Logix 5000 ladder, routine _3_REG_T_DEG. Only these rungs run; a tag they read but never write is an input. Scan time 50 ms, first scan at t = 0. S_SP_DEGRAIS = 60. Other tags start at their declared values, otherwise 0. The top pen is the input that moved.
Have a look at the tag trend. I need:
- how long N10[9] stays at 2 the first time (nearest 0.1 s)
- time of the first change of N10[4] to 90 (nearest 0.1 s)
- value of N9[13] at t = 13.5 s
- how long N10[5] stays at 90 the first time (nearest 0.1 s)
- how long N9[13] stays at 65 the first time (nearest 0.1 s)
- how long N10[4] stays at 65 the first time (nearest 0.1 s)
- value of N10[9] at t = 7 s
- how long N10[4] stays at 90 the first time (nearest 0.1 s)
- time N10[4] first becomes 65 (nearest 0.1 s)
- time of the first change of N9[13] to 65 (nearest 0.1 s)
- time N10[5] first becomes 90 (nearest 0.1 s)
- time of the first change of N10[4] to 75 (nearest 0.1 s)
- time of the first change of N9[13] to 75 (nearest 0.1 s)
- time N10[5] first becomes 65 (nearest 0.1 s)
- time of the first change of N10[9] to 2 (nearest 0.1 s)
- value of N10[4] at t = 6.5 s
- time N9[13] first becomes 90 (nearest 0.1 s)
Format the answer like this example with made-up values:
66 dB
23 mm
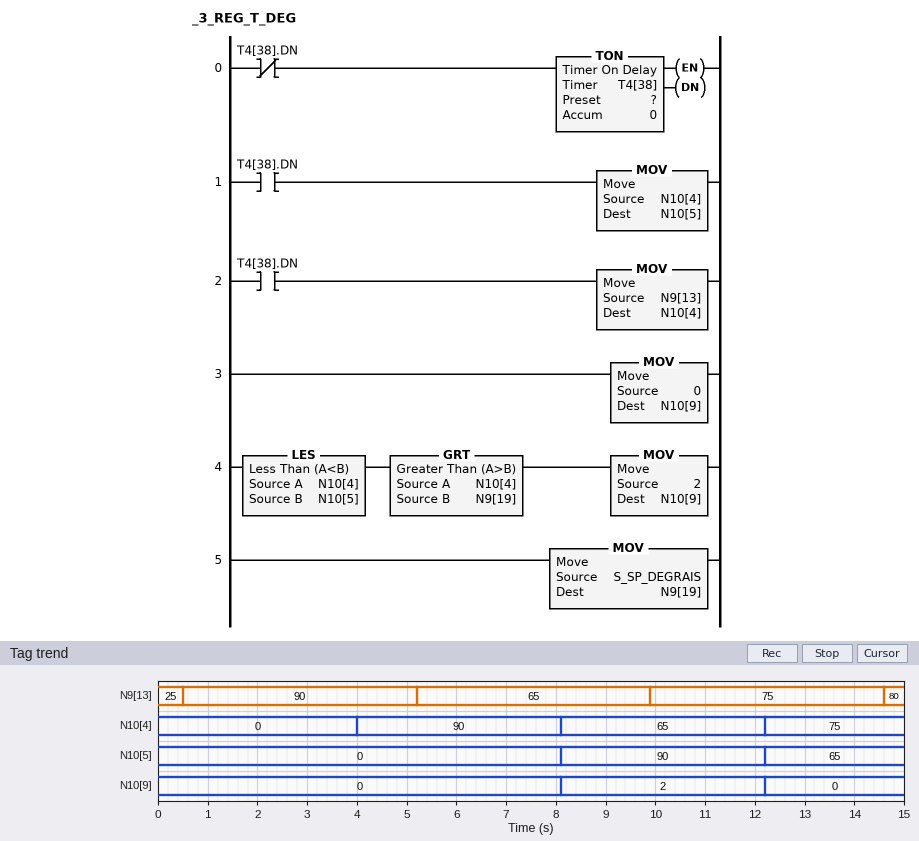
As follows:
4.1 s
4.0 s
75
4.1 s
4.7 s
4.1 s
0
4.1 s
8.1 s
5.2 s
8.1 s
12.2 s
9.9 s
12.2 s
8.1 s
90
0.5 s
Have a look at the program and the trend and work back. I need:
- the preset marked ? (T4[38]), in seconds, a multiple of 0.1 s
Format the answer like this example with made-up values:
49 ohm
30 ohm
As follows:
4.0 s
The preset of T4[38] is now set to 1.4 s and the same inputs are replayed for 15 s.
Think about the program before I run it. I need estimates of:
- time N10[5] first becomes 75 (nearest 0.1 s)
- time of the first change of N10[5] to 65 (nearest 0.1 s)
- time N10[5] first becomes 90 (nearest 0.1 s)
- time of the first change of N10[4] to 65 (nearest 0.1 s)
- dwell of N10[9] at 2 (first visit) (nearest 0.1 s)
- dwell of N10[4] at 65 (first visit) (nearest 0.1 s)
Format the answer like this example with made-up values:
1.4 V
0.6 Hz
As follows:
11.9 s
7.4 s
2.9 s
5.9 s
1.5 s
4.5 s
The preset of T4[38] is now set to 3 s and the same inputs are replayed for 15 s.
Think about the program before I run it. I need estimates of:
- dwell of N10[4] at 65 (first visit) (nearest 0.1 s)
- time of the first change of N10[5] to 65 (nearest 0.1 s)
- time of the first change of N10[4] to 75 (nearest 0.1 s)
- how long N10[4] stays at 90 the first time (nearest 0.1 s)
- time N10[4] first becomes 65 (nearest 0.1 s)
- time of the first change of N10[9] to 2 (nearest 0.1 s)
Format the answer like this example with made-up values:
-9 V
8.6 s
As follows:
6.2 s
9.2 s
12.3 s
3.1 s
6.1 s
6.1 s
